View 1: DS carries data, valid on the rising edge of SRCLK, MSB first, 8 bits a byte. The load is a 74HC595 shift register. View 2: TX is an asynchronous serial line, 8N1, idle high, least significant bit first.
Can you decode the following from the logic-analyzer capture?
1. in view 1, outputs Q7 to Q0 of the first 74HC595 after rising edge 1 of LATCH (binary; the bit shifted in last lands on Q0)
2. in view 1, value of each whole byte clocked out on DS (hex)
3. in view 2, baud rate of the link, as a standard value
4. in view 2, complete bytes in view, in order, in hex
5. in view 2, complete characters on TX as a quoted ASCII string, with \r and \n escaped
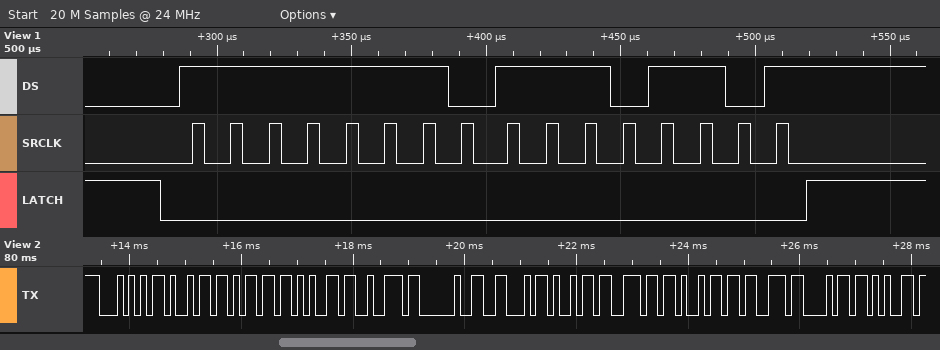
11101101
FE ED
9600 baud
54 69 6D 65 72 20 46 69 6E 69 73 68 65
"Timer Finishe"
